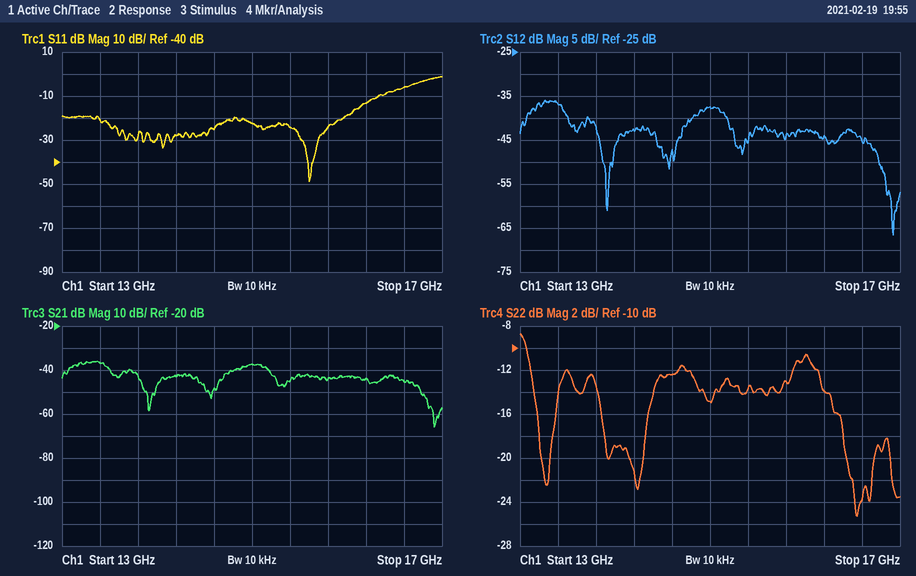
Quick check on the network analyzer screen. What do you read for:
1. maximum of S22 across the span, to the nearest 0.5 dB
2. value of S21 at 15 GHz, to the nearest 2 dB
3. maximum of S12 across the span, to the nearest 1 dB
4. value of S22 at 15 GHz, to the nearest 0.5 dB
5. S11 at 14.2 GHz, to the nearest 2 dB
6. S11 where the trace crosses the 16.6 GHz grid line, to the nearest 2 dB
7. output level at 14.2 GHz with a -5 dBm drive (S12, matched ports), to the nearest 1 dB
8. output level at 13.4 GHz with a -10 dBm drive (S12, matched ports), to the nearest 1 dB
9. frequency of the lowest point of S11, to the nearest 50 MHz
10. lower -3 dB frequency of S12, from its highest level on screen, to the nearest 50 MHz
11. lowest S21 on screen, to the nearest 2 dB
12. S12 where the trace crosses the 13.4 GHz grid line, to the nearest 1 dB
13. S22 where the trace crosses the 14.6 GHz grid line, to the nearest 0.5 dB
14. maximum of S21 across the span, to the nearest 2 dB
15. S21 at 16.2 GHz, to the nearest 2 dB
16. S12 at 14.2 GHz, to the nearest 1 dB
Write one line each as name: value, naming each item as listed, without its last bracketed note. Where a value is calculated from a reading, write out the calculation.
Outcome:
maximum of S22 across the span, to the nearest 0.5 dB: -8.5 dB
value of S21 at 15 GHz, to the nearest 2 dB: -38 dB
maximum of S12 across the span, to the nearest 1 dB: -36 dB
value of S22 at 15 GHz, to the nearest 0.5 dB: -15.0 dB
S11 at 14.2 GHz, to the nearest 2 dB: -28 dB
S11 where the trace crosses the 16.6 GHz grid line, to the nearest 2 dB: -6 dB
output level at 14.2 GHz with a -5 dBm drive (S12, matched ports), to the nearest 1 dB: -5 dBm + (-43 dB) = -48 dBm
output level at 13.4 GHz with a -10 dBm drive (S12, matched ports), to the nearest 1 dB: -10 dBm + (-37 dB) = -47 dBm
frequency of the lowest point of S11, to the nearest 50 MHz: 15.60 GHz
lower -3 dB frequency of S12, from its highest level on screen, to the nearest 50 MHz: 13.10 GHz
lowest S21 on screen, to the nearest 2 dB: -66 dB
S12 where the trace crosses the 13.4 GHz grid line, to the nearest 1 dB: -37 dB
S22 where the trace crosses the 14.6 GHz grid line, to the nearest 0.5 dB: -12.5 dB
maximum of S21 across the span, to the nearest 2 dB: -36 dB
S21 at 16.2 GHz, to the nearest 2 dB: -44 dB
S12 at 14.2 GHz, to the nearest 1 dB: -43 dB
